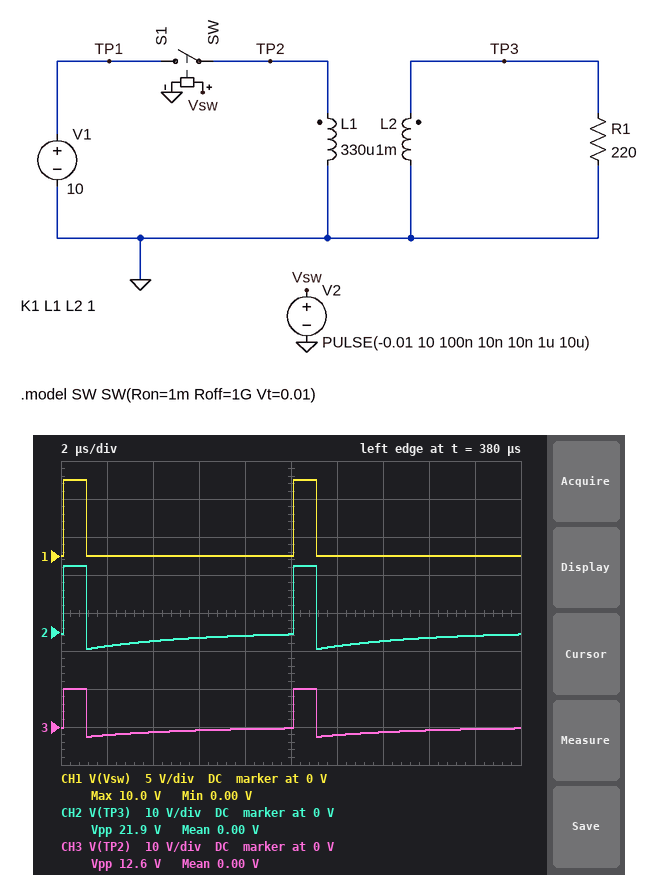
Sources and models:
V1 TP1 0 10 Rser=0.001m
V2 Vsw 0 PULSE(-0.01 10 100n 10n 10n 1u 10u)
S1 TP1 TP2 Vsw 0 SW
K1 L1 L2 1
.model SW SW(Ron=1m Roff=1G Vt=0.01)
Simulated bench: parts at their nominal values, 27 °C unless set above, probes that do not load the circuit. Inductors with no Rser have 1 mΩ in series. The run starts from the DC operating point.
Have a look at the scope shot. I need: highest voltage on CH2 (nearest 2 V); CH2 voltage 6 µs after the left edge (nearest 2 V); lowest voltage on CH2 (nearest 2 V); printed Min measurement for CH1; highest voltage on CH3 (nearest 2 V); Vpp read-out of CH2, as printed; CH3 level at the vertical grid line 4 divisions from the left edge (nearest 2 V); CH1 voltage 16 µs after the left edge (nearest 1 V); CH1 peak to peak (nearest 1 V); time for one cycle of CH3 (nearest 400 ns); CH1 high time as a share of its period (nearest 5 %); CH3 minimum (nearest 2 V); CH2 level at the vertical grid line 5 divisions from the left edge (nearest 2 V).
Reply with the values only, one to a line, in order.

18 V
-2 V
-4 V
0.00 V
10 V
21.9 V
0 V
0 V
10 V
10.0 µs
10 %
-2 V
0 V
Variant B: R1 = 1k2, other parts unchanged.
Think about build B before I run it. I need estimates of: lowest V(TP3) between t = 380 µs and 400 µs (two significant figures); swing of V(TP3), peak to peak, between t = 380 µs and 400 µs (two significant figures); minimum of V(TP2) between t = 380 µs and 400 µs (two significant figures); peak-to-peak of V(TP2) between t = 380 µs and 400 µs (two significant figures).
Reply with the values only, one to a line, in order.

-21 V
39 V
-12 V
22 V
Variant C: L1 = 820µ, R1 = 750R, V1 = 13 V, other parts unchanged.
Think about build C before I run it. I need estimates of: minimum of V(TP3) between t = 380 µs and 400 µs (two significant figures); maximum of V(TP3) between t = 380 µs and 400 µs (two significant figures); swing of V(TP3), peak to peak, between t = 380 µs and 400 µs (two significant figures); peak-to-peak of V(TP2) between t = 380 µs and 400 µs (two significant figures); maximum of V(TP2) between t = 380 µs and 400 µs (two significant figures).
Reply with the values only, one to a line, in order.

-11 V
14 V
25 V
23 V
13 V
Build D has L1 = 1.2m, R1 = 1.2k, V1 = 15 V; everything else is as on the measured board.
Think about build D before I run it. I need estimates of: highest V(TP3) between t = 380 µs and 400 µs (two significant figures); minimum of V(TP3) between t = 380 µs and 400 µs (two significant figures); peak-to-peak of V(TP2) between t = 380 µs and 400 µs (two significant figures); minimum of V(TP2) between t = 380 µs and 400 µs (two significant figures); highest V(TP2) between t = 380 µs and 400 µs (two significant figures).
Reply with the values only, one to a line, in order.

14 V
-17 V
33 V
-18 V
15 V
